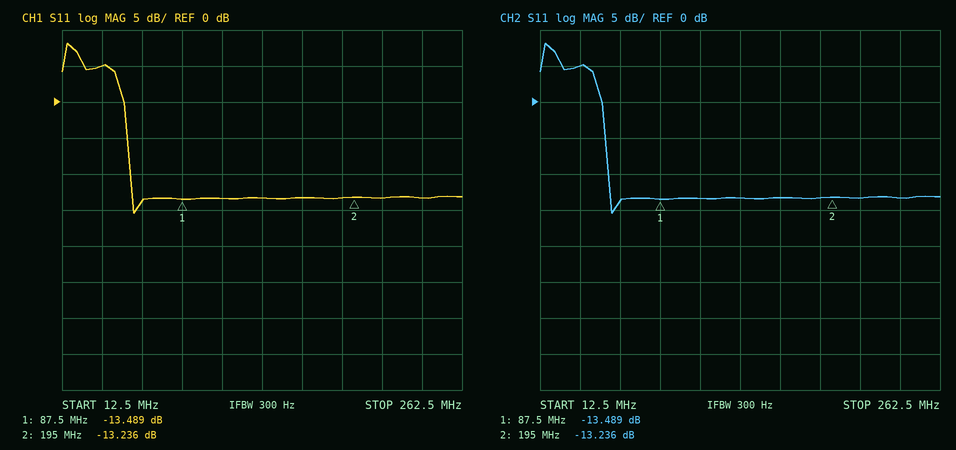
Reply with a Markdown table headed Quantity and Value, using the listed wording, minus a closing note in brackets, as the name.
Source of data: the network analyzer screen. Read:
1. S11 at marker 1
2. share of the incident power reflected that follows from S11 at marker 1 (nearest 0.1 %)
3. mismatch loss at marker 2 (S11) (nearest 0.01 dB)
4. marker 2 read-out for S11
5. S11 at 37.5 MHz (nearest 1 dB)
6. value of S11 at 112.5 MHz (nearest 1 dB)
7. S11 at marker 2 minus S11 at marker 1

| Quantity | Value |
|---|---|
| S11 at marker 1 | -13.489 dB |
| share of the incident power reflected that follows from S11 at marker 1 | 4.5 % |
| mismatch loss at marker 2 (S11) | 0.21 dB |
| marker 2 read-out for S11 | -13.236 dB |
| S11 at 37.5 MHz | 5 dB |
| value of S11 at 112.5 MHz | -13 dB |
| S11 at marker 2 minus S11 at marker 1 | 0.253 dB |
